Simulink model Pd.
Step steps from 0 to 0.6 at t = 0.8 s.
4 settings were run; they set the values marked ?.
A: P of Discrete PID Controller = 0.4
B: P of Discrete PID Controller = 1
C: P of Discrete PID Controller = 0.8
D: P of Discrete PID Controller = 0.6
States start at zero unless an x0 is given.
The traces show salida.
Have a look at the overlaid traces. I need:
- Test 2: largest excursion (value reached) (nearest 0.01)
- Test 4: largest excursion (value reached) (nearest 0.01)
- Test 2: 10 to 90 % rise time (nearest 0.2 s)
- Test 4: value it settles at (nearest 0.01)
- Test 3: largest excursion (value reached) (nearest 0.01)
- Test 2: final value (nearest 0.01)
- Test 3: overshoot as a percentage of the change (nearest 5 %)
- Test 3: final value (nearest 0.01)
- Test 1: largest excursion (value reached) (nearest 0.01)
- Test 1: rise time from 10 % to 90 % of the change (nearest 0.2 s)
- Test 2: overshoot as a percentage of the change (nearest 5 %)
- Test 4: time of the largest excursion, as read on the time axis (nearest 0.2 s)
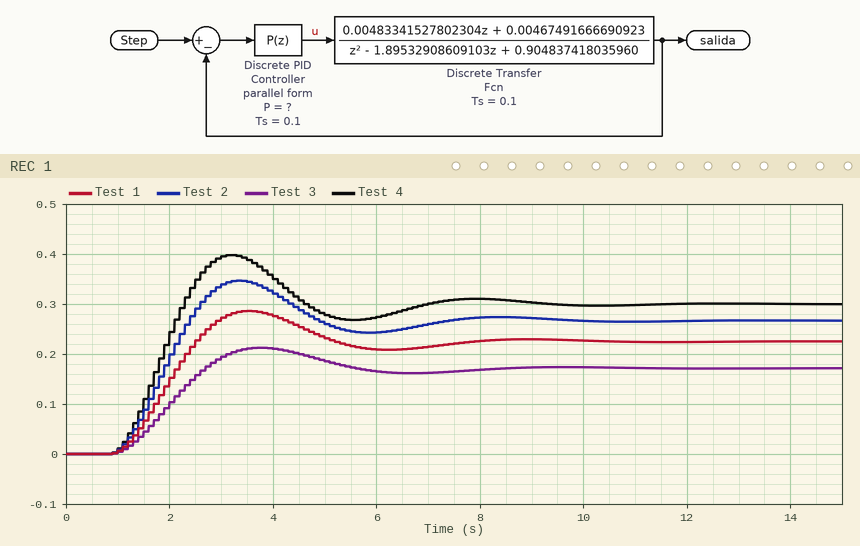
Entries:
0.35
0.40
1.0 s
0.30
0.21
0.27
25 %
0.17
0.29
1.2 s
30 %
3.2 s
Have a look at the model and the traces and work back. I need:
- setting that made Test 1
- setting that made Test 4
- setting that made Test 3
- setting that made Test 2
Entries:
D
B
A
C
